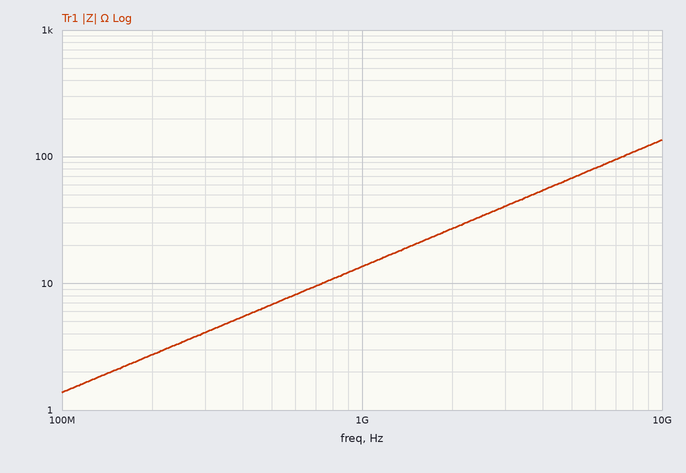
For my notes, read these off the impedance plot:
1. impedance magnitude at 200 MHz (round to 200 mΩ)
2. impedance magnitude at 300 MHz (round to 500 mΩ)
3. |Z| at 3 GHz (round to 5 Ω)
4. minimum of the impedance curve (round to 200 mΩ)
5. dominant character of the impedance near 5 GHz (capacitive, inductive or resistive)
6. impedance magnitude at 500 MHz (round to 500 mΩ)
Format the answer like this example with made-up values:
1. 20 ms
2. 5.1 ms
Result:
1. 2.8 Ω
2. 4.0 Ω
3. 40 Ω
4. 1.4 Ω
5. inductive
6. 7.0 Ω
